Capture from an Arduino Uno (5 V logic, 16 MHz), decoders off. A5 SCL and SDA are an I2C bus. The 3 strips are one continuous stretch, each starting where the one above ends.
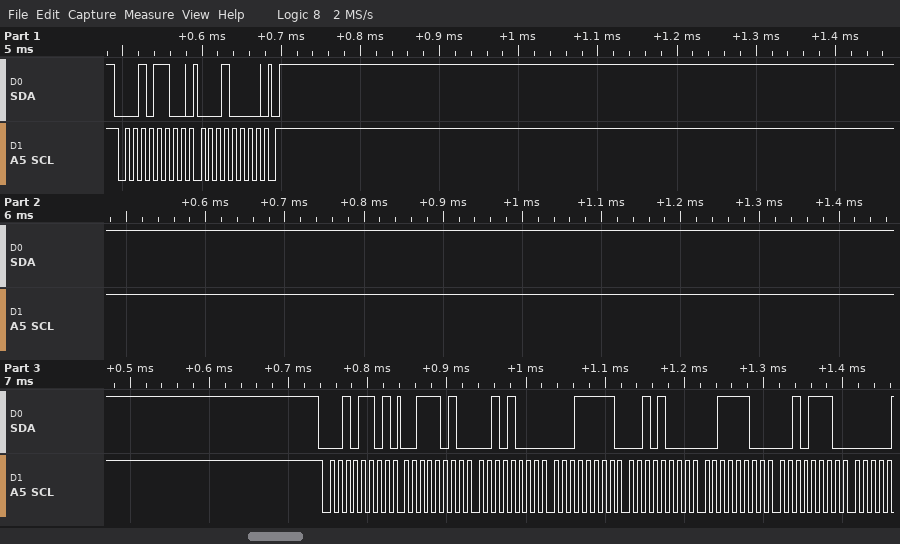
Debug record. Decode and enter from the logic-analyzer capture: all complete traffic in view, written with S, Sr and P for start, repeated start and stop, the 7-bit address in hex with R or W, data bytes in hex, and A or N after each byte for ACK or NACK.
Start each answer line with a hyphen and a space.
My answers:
- S 16W A 10 A P S 16R A 3A A 28 A 1F A 28 A 3C A 2E A
